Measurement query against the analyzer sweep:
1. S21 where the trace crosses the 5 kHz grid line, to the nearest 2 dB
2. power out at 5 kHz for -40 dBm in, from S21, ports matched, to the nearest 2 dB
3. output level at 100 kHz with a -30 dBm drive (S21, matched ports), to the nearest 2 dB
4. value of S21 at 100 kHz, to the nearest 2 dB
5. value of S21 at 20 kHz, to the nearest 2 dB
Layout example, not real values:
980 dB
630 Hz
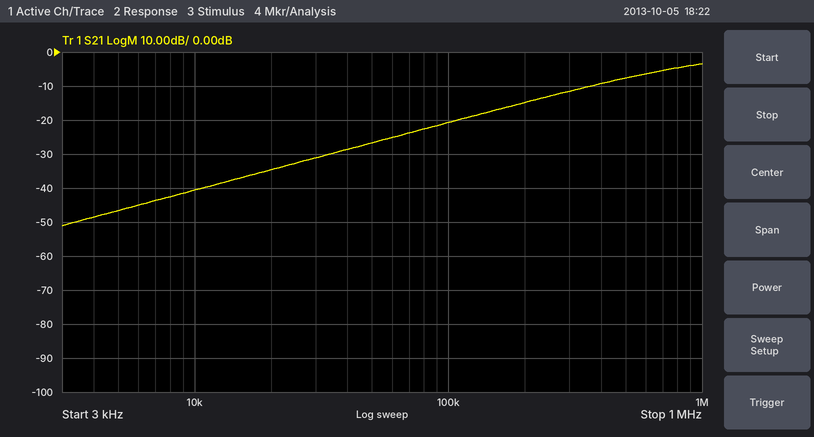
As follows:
-46 dB
-86 dBm
-50 dBm
-20 dB
-34 dB
